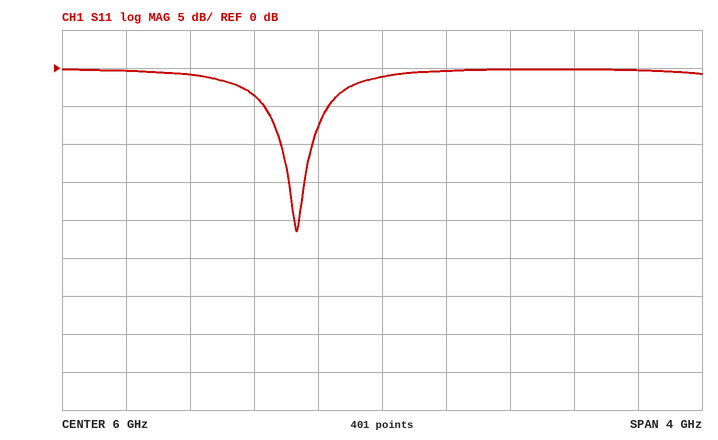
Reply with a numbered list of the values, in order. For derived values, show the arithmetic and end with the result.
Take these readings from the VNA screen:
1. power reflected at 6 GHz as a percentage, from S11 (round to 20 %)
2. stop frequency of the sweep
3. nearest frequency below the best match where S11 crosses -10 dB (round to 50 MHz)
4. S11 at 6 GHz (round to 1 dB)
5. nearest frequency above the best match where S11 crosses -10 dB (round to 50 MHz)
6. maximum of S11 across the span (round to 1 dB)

1. 10^(-1/10) ≈ 79.4 %, so 80 % to the nearest 20 %
2. 8 GHz
3. 5.35 GHz
4. -1 dB
5. 5.55 GHz
6. 0 dB
